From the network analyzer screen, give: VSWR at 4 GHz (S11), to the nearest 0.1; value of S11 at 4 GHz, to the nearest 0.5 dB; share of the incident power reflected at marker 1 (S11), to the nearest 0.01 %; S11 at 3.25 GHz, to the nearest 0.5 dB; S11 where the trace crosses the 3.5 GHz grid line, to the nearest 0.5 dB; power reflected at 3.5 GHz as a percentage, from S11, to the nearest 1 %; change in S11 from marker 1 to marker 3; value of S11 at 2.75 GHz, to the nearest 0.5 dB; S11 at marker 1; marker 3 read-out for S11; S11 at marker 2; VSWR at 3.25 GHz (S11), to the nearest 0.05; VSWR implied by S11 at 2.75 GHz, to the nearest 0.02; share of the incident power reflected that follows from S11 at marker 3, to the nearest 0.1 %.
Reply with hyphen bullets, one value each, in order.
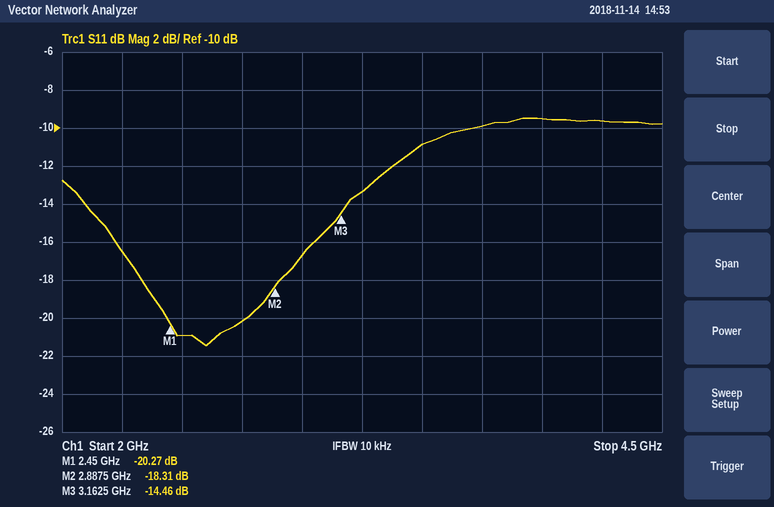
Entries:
- 2.0
- -9.5 dB
- 0.94 %
- -13.5 dB
- -11.0 dB
- 8 %
- 5.81 dB
- -20.0 dB
- -20.27 dB
- -14.46 dB
- -18.31 dB
- 1.55
- 1.22
- 3.6 %
